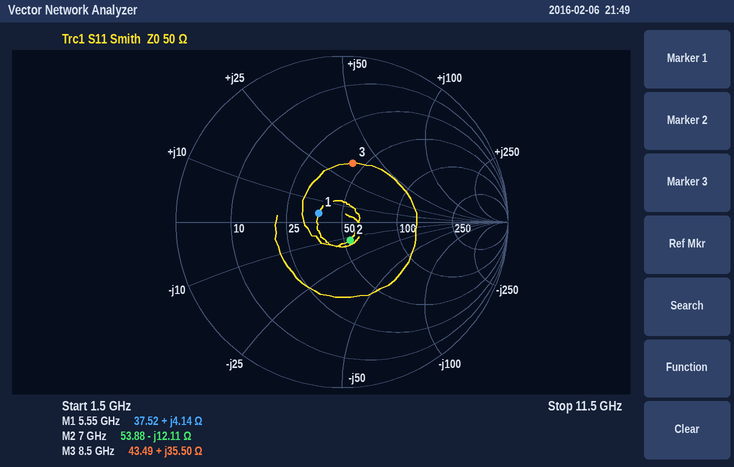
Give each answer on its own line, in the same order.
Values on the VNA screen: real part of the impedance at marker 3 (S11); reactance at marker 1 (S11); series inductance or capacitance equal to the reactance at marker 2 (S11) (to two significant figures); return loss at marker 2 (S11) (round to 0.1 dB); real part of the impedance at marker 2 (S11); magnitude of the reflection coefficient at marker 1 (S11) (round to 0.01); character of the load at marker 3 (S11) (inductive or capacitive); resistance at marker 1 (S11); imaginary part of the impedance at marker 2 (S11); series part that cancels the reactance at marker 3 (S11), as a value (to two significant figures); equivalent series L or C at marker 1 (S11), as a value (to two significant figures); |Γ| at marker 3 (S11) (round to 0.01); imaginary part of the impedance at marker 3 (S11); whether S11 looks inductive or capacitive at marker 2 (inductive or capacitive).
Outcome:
43.49 Ω
+4.14 Ω
1.9 pF
18.3 dB
53.88 Ω
0.15
inductive
37.52 Ω
-12.11 Ω
530 fF
120 pH
0.36
+35.50 Ω
capacitive
